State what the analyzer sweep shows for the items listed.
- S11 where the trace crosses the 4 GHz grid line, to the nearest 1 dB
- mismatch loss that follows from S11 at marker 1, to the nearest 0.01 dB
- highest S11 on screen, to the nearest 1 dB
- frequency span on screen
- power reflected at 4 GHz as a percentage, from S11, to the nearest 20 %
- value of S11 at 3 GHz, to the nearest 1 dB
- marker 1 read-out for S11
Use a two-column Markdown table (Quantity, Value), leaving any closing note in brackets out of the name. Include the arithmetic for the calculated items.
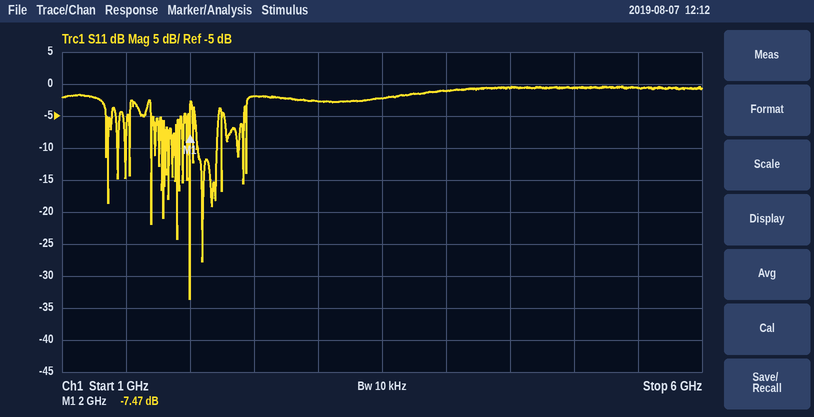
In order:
| Quantity | Value |
|---|---|
| S11 where the trace crosses the 4 GHz grid line, to the nearest 1 dB | -1 dB |
| mismatch loss that follows from S11 at marker 1, to the nearest 0.01 dB | −10 log10(1 − 10^(-7.47/10)) ≈ 0.86 dB |
| highest S11 on screen, to the nearest 1 dB | 0 dB |
| frequency span on screen | 5 GHz |
| power reflected at 4 GHz as a percentage, from S11, to the nearest 20 % | 10^(-1/10) ≈ 79.4 %, so 80 % to the nearest 20 % |
| value of S11 at 3 GHz, to the nearest 1 dB | -3 dB |
| marker 1 read-out for S11 | -7.47 dB |
